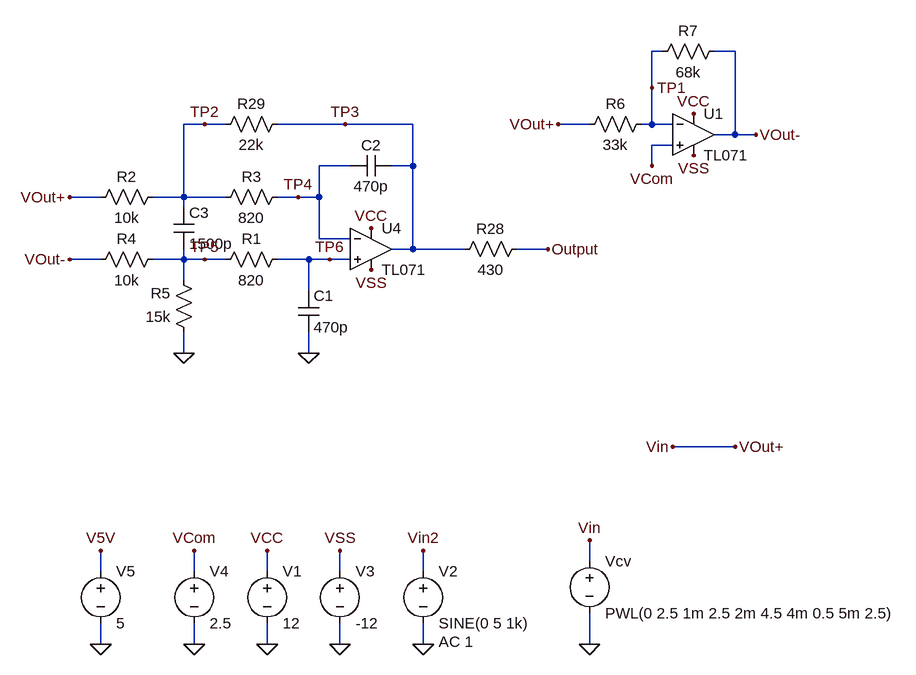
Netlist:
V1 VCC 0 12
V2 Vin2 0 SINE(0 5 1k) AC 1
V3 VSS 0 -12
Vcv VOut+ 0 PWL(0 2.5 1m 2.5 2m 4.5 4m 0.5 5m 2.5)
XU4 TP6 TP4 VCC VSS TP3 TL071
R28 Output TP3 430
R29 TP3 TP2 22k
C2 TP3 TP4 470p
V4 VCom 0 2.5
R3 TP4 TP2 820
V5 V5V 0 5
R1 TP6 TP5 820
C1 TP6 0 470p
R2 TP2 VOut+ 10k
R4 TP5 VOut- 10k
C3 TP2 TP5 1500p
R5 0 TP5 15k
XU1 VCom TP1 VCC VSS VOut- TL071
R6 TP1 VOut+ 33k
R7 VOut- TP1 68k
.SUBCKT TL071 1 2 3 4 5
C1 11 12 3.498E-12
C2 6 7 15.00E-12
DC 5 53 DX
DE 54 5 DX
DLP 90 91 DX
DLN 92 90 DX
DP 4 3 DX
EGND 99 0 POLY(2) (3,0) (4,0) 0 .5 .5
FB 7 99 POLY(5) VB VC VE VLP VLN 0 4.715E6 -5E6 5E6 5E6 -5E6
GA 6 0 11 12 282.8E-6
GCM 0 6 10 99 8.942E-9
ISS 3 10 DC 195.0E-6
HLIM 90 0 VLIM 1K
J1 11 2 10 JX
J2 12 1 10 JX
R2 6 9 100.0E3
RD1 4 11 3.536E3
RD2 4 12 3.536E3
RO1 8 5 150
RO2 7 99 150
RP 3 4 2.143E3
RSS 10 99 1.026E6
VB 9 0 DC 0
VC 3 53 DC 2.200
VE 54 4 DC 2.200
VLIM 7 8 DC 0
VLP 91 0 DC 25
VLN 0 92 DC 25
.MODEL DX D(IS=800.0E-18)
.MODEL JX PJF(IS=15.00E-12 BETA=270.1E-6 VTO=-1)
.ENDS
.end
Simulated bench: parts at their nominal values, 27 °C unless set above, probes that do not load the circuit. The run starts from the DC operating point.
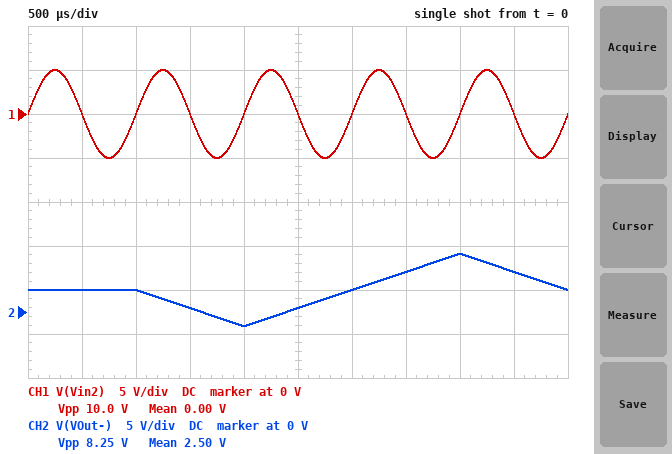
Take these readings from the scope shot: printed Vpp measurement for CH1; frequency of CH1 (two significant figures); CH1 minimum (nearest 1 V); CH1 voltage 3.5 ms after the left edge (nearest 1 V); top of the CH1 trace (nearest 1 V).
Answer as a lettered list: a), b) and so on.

a) 10.0 V
b) 1.0 kHz
c) -5 V
d) 0 V
e) 5 V
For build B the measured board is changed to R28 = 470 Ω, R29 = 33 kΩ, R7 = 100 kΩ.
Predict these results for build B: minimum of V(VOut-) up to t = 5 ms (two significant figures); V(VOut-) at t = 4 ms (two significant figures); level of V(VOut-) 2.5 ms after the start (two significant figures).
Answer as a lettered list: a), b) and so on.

a) -3.6 V
b) 8.6 V
c) -530 mV
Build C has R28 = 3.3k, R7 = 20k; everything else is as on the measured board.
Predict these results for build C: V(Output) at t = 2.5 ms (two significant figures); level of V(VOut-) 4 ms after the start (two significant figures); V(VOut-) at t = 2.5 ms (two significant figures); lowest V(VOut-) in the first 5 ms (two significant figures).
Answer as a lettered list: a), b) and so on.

a) -4.1 V
b) 3.7 V
c) 1.9 V
d) 1.3 V
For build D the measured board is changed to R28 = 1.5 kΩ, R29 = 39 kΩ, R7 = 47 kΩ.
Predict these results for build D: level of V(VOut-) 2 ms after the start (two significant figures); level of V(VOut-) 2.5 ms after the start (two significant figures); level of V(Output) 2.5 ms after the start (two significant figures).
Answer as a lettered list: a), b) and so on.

a) -350 mV
b) 1.1 V
c) -10 V
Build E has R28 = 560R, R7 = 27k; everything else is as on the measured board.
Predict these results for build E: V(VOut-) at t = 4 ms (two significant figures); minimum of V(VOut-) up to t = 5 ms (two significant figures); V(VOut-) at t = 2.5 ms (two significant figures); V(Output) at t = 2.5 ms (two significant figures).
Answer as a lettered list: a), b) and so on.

a) 4.1 V
b) 860 mV
c) 1.7 V
d) -4.6 V
